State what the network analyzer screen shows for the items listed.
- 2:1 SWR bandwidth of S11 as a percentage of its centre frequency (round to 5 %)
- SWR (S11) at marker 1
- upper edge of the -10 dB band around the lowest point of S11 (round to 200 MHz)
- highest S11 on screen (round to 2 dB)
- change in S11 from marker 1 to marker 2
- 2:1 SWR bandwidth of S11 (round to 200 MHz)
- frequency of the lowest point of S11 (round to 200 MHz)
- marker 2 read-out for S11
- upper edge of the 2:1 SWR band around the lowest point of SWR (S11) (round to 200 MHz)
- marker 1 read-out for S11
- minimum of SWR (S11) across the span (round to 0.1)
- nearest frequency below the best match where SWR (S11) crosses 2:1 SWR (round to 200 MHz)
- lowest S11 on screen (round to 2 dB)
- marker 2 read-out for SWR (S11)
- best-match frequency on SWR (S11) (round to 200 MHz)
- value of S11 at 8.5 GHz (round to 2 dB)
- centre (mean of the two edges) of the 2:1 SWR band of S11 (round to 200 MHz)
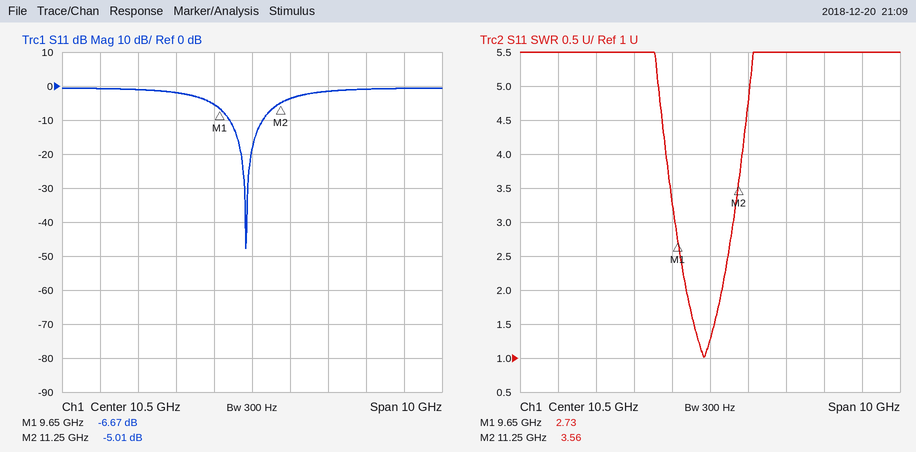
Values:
10 %
2.73
10.8 GHz
0 dB
1.66 dB
1.0 GHz
10.4 GHz
-5.01 dB
10.8 GHz
-6.67 dB
1.0
9.8 GHz
-48 dB
3.56
10.4 GHz
-2 dB
10.4 GHz
